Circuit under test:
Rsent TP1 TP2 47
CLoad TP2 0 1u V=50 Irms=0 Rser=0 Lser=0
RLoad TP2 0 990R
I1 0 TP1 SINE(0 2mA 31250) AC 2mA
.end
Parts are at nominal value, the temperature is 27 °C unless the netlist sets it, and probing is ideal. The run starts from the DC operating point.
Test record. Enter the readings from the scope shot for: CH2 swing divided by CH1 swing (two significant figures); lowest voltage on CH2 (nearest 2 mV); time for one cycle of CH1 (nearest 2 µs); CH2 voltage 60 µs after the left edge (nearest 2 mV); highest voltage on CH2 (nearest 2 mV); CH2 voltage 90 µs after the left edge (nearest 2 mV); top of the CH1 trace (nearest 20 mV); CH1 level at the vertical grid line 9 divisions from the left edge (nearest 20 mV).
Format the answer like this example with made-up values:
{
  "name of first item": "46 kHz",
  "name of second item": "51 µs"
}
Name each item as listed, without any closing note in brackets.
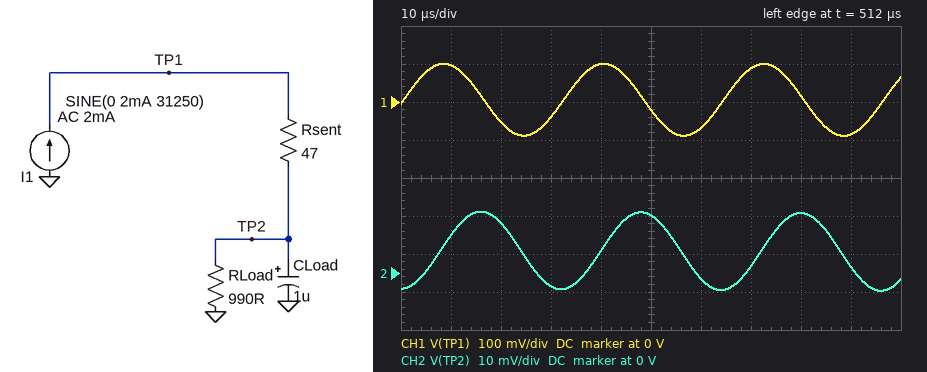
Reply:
{
  "CH2 swing divided by CH1 swing": "0.11",
  "lowest voltage on CH2": "-4 mV",
  "time for one cycle of CH1": "32 µs",
  "CH2 voltage 60 µs after the left edge": "-2 mV",
  "highest voltage on CH2": "16 mV",
  "CH2 voltage 90 µs after the left edge": "2 mV",
  "top of the CH1 trace": "100 mV",
  "CH1 level at the vertical grid line 9 divisions from the left edge": "-80 mV"
}
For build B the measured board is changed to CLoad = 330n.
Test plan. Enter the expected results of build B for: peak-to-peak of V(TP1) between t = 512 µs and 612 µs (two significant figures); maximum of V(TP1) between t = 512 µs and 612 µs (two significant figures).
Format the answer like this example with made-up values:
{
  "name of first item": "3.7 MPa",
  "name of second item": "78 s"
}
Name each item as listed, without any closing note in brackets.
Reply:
{
  "peak-to-peak of V(TP1) between t = 512 µs and 612 µs": "200 mV",
  "maximum of V(TP1) between t = 512 µs and 612 µs": "110 mV"
}
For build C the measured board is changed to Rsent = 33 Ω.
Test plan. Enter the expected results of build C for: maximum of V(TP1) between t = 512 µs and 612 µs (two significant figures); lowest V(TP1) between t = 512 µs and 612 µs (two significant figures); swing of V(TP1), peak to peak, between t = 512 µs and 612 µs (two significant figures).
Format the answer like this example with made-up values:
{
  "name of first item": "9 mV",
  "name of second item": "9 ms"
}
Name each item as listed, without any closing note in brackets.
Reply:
{
  "maximum of V(TP1) between t = 512 µs and 612 µs": "73 mV",
  "lowest V(TP1) between t = 512 µs and 612 µs": "-61 mV",
  "swing of V(TP1), peak to peak, between t = 512 µs and 612 µs": "130 mV"
}
